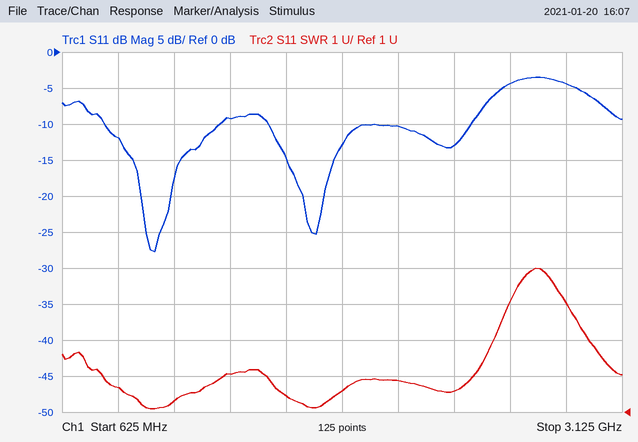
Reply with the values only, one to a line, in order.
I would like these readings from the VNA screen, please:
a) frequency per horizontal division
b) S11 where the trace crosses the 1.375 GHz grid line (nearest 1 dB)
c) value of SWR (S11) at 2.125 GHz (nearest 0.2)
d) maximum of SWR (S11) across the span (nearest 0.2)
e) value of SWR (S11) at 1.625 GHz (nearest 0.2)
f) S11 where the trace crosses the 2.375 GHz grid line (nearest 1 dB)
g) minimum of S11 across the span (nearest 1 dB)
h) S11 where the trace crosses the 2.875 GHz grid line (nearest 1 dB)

250 MHz
-9 dB
1.8
5.0
1.4
-13 dB
-28 dB
-4 dB
